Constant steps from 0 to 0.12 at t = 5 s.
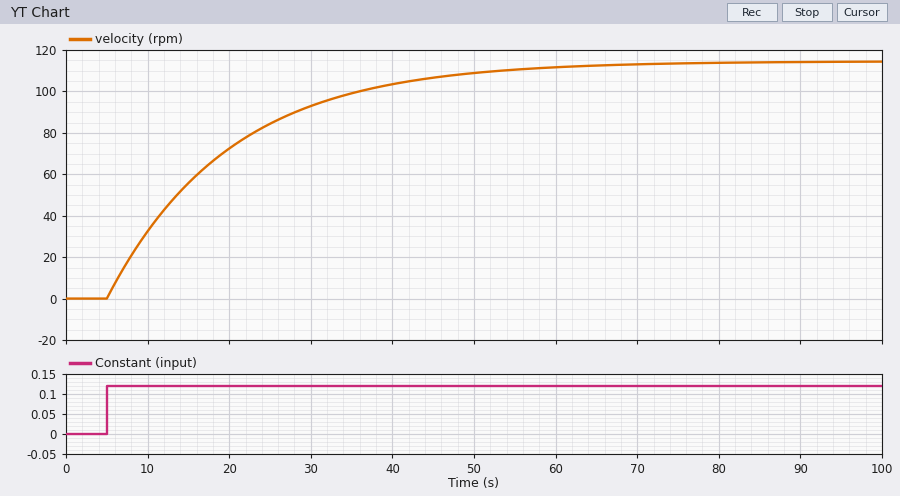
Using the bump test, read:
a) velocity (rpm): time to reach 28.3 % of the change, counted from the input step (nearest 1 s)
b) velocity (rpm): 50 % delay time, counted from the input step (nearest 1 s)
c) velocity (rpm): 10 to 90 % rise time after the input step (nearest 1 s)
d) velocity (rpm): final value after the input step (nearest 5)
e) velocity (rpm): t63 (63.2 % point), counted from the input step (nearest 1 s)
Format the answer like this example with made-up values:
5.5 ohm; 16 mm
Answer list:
5 s; 10 s; 33 s; 115; 15 s
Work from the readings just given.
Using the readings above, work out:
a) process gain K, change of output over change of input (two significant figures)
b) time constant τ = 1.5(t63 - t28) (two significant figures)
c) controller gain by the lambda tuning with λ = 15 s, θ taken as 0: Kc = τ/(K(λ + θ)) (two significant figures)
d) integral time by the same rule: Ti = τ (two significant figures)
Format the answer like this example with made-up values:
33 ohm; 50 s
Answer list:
960; 15 s; 0.0010; 15 s
